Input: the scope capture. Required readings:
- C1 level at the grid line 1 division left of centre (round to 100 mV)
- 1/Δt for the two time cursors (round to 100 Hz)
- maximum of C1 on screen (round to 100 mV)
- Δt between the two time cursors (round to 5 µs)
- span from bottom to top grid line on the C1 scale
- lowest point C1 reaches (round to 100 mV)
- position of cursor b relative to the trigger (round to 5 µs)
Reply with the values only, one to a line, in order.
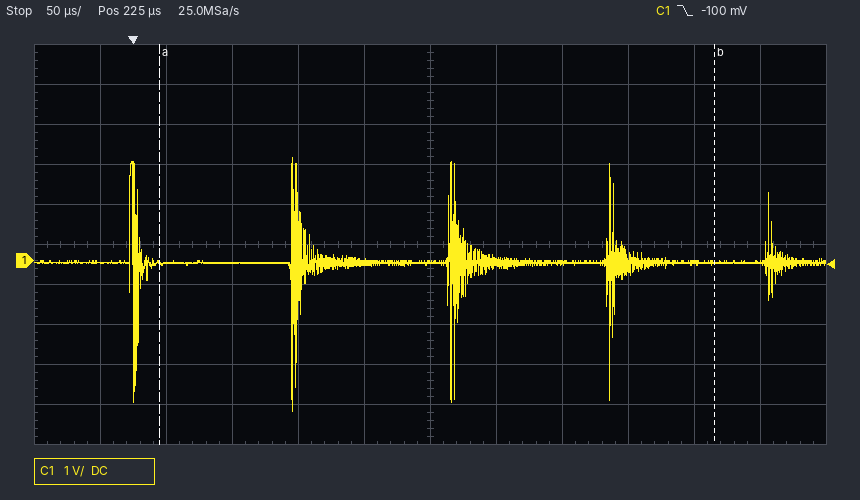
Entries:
0.0 V
2.4 kHz
2.6 V
420 µs
10 V
-3.8 V
+440 µs
